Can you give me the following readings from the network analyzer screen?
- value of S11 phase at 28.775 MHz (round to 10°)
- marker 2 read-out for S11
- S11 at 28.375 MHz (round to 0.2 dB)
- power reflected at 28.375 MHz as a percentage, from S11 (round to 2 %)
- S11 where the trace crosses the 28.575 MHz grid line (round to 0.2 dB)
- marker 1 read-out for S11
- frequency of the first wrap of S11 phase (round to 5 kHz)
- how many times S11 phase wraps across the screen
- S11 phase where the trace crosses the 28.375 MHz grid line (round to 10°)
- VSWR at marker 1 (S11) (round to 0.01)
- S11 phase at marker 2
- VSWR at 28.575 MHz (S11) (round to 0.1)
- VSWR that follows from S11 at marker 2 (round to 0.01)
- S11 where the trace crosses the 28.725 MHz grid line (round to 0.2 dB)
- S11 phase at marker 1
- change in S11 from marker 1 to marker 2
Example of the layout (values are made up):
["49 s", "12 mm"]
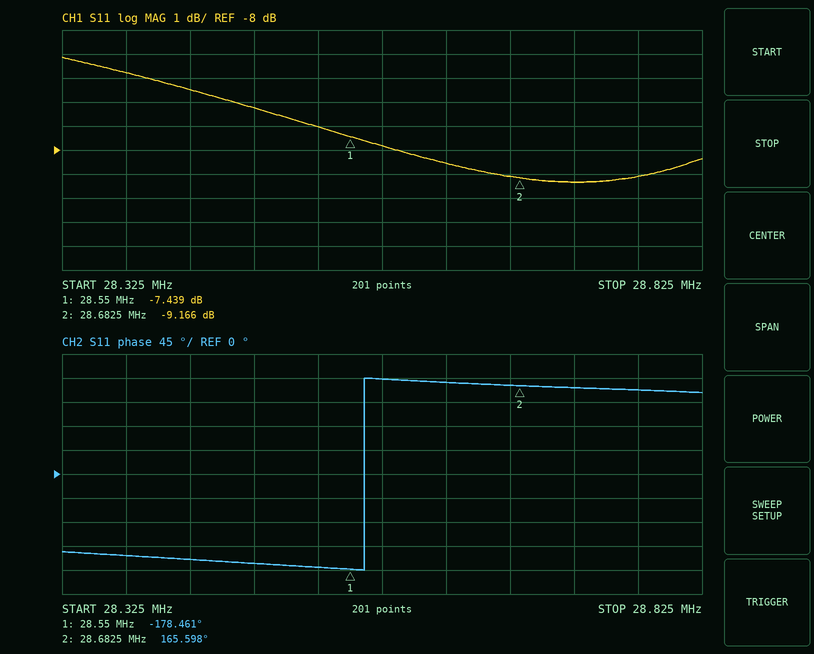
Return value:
["160°", "-9.166 dB", "-4.8 dB", "34 %", "-7.8 dB", "-7.439 dB", "28.560 MHz", "1", "-150°", "2.48", "165.598°", "2.4", "2.07", "-9.4 dB", "-178.461°", "-1.727 dB"]
